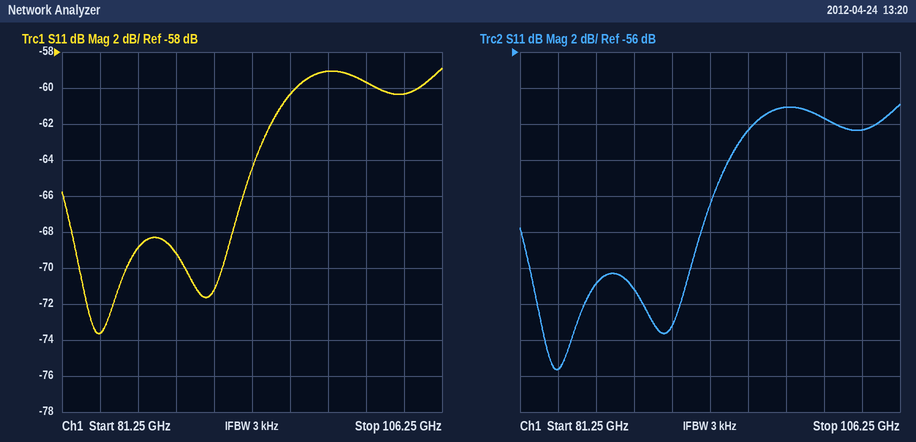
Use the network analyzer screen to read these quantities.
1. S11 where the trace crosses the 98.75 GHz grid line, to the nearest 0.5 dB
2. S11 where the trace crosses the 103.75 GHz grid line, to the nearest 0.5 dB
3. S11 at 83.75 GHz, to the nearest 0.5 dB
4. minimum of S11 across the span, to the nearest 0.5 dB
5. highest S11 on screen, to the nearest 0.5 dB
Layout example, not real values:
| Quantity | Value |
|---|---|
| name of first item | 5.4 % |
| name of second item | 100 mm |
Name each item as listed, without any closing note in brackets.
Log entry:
| Quantity | Value |
|---|---|
| S11 where the trace crosses the 98.75 GHz grid line, to the nearest 0.5 dB | -59.0 dB |
| S11 where the trace crosses the 103.75 GHz grid line, to the nearest 0.5 dB | -60.5 dB |
| S11 at 83.75 GHz, to the nearest 0.5 dB | -73.5 dB |
| minimum of S11 across the span, to the nearest 0.5 dB | -73.5 dB |
| highest S11 on screen, to the nearest 0.5 dB | -59.0 dB |
